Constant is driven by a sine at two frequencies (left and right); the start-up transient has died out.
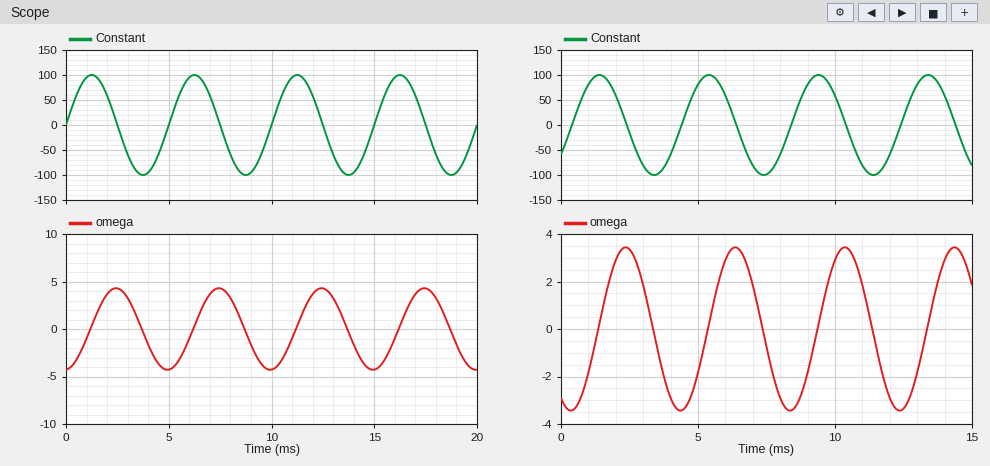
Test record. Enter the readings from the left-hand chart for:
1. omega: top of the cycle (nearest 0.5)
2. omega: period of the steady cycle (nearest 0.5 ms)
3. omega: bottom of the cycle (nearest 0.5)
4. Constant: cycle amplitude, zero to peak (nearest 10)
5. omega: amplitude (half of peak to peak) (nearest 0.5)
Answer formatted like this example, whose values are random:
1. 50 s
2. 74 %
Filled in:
1. 4.5
2. 5.0 ms
3. -4.5
4. 100
5. 4.5
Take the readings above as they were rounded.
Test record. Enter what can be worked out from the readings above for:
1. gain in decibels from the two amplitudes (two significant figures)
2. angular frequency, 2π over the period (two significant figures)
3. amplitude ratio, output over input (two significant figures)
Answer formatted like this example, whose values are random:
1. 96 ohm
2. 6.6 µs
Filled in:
1. -27 dB
2. 1.3 rad/ms
3. 0.045
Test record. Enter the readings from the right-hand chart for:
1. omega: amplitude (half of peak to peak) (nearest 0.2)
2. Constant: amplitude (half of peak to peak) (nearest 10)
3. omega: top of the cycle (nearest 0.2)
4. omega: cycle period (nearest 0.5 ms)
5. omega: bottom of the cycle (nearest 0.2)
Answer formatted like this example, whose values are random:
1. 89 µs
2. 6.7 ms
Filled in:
1. 3.4
2. 100
3. 3.4
4. 4.0 ms
5. -3.4
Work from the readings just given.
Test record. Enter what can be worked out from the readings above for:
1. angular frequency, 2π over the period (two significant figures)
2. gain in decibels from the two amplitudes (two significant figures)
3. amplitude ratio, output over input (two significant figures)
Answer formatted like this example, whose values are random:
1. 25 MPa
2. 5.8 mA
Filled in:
1. 1.6 rad/ms
2. -29 dB
3. 0.034
